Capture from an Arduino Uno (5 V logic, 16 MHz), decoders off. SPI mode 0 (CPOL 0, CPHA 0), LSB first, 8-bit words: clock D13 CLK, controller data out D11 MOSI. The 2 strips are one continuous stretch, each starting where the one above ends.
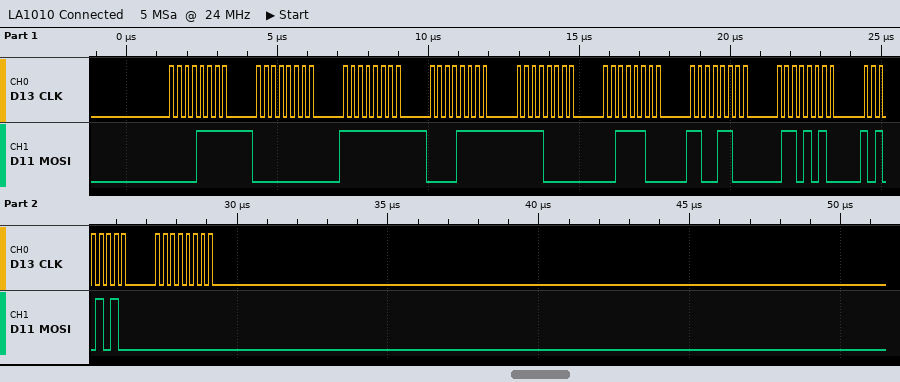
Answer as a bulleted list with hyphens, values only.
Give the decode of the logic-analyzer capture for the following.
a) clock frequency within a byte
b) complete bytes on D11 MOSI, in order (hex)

- 4 MHz
- F0 00 FF F0 0F 3C 33 56 55 00
